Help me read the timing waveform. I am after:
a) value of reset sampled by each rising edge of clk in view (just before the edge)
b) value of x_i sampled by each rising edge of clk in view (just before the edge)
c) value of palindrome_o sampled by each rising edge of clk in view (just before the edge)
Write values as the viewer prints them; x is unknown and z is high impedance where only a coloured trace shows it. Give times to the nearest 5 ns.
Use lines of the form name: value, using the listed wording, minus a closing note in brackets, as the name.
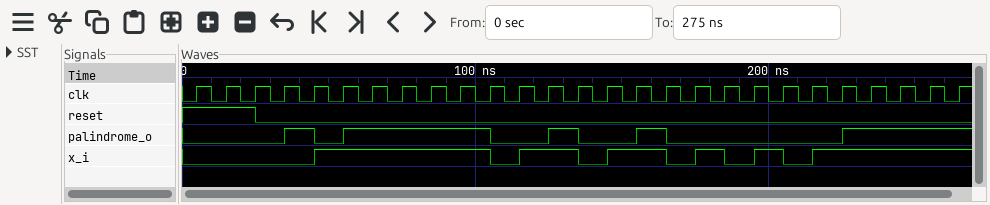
value of reset sampled by each rising edge of clk in view: 1 1 1 0 0 0 0 0 0 0 0 0 0 0 0 0 0 0 0 0 0 0 0 0 0 0 0
value of x_i sampled by each rising edge of clk in view: 0 0 0 0 0 1 1 1 1 1 1 0 1 1 0 1 1 0 1 0 1 0 1 1 1 1 1
value of palindrome_o sampled by each rising edge of clk in view: 0 0 0 0 1 0 1 1 1 1 1 0 0 1 0 0 1 0 0 0 0 0 0 1 1 1 1
